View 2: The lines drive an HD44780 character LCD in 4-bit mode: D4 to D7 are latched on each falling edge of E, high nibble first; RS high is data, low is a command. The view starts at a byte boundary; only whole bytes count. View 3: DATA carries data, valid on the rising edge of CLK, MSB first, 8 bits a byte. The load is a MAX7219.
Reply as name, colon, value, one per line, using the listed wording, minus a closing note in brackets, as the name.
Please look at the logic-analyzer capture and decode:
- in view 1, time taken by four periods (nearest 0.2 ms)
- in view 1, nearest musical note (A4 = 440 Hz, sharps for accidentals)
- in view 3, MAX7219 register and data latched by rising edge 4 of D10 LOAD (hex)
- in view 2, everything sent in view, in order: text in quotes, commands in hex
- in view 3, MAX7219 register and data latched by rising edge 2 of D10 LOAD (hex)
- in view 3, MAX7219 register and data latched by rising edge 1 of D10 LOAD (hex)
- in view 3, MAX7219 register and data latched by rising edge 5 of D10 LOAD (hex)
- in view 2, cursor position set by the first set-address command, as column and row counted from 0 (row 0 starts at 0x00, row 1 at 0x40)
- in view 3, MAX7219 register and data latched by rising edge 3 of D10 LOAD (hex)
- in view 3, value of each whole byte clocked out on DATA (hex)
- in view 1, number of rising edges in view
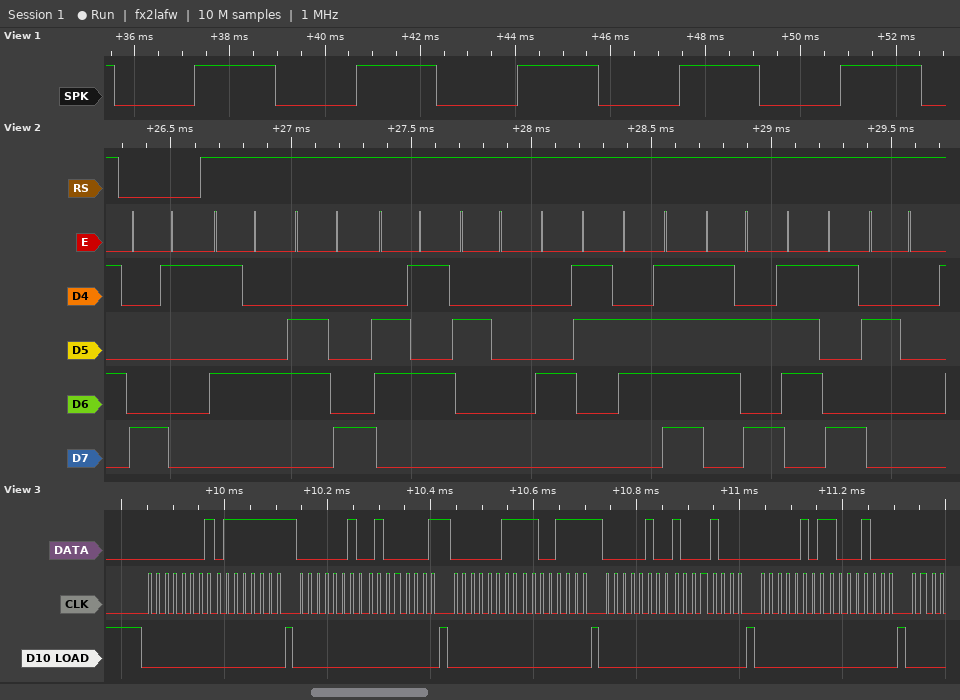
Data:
in view 1, time taken by four periods: 13.6 ms
in view 1, nearest musical note: D4
in view 3, MAX7219 register and data latched by rising edge 4 of D10 LOAD: register 0x4, data 0x88
in view 2, everything sent in view, in order: text in quotes, commands in hex: 0x81 "The Cozy "
in view 3, MAX7219 register and data latched by rising edge 2 of D10 LOAD: register 0x2, data 0x41
in view 3, MAX7219 register and data latched by rising edge 1 of D10 LOAD: register 0x1, data 0x7F
in view 3, MAX7219 register and data latched by rising edge 5 of D10 LOAD: register 0x5, data 0x88
in view 2, cursor position set by the first set-address command, as column and row counted from 0: column 1, row 0
in view 3, MAX7219 register and data latched by rising edge 3 of D10 LOAD: register 0x3, data 0xCF
in view 3, value of each whole byte clocked out on DATA: 0x01 0x7F 0x02 0x41 0x03 0xCF 0x04 0x88 0x05 0x88
in view 1, number of rising edges in view: 5
